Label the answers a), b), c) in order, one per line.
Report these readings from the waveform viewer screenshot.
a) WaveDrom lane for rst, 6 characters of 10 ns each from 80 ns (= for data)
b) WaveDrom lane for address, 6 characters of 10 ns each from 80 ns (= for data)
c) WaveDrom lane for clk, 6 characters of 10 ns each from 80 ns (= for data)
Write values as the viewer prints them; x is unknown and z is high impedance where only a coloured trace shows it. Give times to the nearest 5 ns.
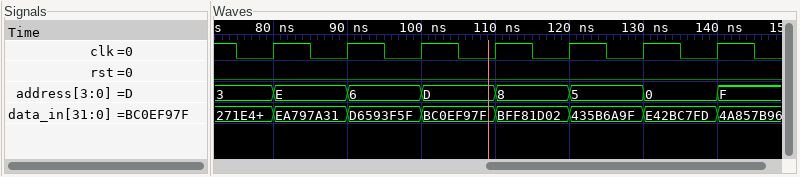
a) {name: 'rst', wave: '0.....'}
b) {name: 'address', wave: '======', data: 'E 6 D 8 5 0'}
c) {name: 'clk', wave: 'p.....'}
